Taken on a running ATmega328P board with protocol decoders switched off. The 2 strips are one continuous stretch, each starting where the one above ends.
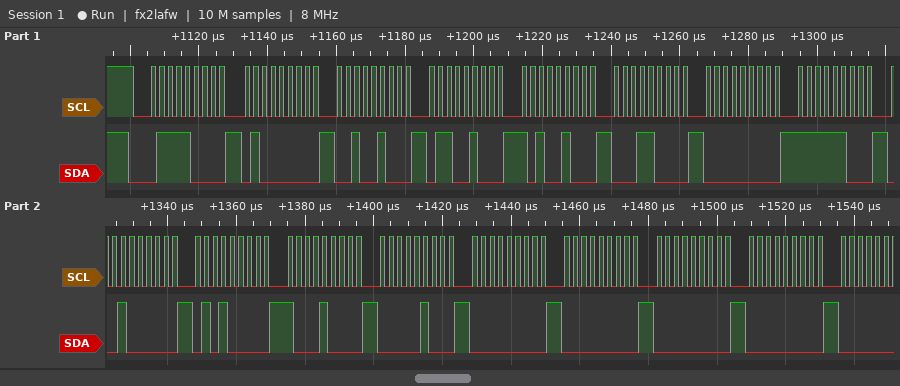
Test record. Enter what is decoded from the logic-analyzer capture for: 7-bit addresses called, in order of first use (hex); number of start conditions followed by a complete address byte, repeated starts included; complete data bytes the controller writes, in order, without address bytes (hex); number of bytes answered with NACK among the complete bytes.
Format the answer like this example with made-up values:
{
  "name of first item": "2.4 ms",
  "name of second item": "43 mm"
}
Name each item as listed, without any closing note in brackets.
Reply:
{
  "7-bit addresses called, in order of first use": "0x3C",
  "number of start conditions followed by a complete address byte, repeated starts included": "1",
  "complete data bytes the controller writes, in order, without address bytes": "40 24 64 A4 18 00 FC 20 50 88 04 00 00 00 00",
  "number of bytes answered with NACK among the complete bytes": "0"
}
